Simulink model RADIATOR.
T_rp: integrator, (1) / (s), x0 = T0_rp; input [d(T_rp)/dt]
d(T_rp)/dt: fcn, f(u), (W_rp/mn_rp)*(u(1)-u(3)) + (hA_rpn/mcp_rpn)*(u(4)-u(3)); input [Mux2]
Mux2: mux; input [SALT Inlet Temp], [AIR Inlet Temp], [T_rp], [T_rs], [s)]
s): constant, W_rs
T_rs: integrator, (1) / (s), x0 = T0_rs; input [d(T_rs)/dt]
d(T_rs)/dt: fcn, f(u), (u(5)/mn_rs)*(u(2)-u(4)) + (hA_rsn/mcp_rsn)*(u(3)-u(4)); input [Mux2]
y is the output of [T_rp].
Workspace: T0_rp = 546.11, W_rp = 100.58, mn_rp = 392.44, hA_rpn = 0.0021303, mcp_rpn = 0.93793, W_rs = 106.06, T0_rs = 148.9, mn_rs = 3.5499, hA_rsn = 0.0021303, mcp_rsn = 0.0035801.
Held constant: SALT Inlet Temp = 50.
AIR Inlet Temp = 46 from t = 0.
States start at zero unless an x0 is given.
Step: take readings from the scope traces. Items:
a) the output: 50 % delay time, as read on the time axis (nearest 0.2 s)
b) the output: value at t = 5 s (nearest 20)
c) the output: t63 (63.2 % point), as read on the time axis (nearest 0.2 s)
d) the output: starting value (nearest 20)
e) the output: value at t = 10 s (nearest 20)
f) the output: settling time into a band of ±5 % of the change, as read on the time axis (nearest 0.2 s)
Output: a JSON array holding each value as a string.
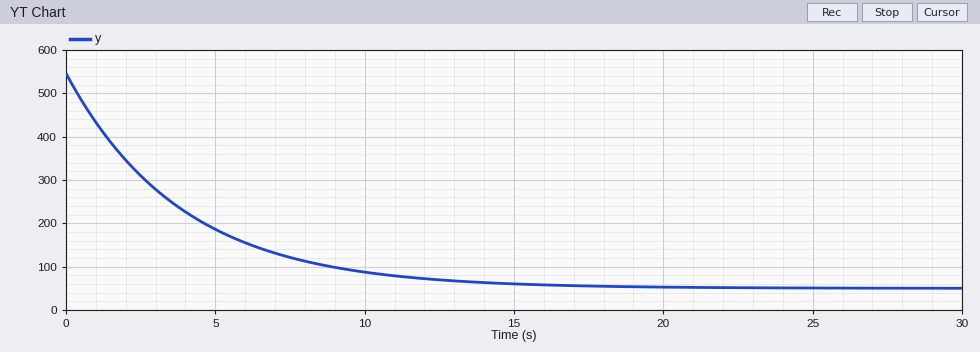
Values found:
["2.6 s", "180", "3.8 s", "540", "80", "11.6 s"]
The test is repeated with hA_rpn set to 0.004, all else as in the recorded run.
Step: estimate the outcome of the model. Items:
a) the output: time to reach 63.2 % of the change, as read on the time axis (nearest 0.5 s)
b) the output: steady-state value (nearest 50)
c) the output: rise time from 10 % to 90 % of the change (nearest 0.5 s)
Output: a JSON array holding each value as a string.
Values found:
["4.0 s", "50", "8.5 s"]
